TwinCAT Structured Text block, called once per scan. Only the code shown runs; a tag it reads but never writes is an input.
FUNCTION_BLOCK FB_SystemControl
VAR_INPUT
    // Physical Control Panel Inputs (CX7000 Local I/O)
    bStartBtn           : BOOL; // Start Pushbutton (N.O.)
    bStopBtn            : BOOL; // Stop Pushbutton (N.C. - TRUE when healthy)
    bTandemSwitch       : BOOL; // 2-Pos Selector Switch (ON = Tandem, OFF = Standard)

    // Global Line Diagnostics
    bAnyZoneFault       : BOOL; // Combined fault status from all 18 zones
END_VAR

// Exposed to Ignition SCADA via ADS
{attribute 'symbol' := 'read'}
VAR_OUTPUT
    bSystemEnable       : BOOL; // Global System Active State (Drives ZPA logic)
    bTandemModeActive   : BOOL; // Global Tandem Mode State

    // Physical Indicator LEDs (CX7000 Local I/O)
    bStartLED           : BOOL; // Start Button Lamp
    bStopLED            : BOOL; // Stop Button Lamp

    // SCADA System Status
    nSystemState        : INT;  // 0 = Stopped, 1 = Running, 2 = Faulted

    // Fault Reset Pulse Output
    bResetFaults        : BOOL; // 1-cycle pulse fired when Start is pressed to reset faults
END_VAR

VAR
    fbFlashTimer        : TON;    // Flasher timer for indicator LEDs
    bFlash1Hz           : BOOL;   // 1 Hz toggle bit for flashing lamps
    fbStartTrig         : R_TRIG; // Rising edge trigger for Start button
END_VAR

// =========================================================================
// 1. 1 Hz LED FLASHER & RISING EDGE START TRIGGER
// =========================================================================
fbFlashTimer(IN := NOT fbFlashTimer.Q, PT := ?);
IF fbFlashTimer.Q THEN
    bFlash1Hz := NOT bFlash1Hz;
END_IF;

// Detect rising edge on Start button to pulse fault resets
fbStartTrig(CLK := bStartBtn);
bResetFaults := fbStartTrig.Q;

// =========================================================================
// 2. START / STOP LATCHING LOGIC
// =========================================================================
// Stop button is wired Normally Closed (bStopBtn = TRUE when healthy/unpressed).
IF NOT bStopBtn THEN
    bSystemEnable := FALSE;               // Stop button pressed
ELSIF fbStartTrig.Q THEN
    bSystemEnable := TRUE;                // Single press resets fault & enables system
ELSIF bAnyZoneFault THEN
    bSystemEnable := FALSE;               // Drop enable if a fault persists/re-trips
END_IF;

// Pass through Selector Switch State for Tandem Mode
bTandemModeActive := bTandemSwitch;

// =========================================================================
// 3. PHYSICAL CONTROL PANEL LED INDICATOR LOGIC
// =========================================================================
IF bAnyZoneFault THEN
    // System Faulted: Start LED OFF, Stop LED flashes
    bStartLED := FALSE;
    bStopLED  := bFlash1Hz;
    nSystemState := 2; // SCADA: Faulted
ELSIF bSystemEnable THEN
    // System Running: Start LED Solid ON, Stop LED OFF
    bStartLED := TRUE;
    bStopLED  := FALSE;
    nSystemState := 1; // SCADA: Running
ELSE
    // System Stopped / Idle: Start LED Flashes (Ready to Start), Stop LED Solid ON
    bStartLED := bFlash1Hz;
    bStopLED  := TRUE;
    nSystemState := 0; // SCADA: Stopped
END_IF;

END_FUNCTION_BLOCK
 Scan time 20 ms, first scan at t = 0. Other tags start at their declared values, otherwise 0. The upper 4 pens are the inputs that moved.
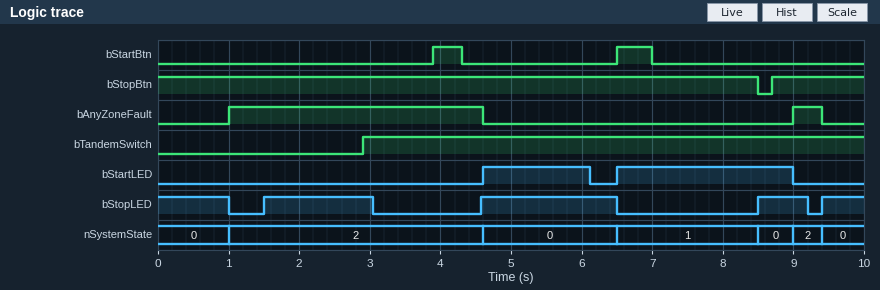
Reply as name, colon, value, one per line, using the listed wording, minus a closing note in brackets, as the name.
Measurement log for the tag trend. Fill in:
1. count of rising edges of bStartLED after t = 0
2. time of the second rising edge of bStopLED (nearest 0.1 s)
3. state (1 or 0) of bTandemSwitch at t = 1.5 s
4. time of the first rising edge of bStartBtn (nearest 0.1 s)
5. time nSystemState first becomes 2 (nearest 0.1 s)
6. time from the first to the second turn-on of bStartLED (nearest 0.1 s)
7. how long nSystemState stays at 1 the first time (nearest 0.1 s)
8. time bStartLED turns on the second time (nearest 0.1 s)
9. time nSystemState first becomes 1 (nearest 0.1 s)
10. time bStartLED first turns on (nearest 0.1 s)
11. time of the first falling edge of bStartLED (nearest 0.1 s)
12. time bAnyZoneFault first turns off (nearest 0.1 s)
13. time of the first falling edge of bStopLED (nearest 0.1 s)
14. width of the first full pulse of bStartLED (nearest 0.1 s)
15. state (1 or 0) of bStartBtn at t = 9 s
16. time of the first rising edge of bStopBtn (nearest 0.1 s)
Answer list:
count of rising edges of bStartLED after t = 0: 2
time of the second rising edge of bStopLED: 4.6 s
state (1 or 0) of bTandemSwitch at t = 1.5 s: 0
time of the first rising edge of bStartBtn: 3.9 s
time nSystemState first becomes 2: 1.0 s
time from the first to the second turn-on of bStartLED: 1.9 s
how long nSystemState stays at 1 the first time: 2.0 s
time bStartLED turns on the second time: 6.5 s
time nSystemState first becomes 1: 6.5 s
time bStartLED first turns on: 4.6 s
time of the first falling edge of bStartLED: 6.1 s
time bAnyZoneFault first turns off: 4.6 s
time of the first falling edge of bStopLED: 1.0 s
width of the first full pulse of bStartLED: 1.5 s
state (1 or 0) of bStartBtn at t = 9 s: 0
time of the first rising edge of bStopBtn: 8.7 s
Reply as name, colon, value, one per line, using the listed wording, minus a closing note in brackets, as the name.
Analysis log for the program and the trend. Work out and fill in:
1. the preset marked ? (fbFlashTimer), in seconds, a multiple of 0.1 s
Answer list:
the preset marked ? (fbFlashTimer), in seconds, a multiple of 0.1 s: 1.5 s
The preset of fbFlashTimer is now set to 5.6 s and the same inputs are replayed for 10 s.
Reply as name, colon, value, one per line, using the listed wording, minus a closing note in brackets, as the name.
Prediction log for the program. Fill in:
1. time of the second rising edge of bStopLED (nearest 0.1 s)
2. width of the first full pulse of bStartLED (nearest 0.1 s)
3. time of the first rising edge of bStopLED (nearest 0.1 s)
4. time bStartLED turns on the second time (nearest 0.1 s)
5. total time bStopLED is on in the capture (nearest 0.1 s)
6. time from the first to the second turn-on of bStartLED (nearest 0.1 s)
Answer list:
time of the second rising edge of bStopLED: 8.5 s
width of the first full pulse of bStartLED: 3.4 s
time of the first rising edge of bStopLED: 4.6 s
time bStartLED turns on the second time: 9.4 s
total time bStopLED is on in the capture: 4.4 s
time from the first to the second turn-on of bStartLED: 3.8 s
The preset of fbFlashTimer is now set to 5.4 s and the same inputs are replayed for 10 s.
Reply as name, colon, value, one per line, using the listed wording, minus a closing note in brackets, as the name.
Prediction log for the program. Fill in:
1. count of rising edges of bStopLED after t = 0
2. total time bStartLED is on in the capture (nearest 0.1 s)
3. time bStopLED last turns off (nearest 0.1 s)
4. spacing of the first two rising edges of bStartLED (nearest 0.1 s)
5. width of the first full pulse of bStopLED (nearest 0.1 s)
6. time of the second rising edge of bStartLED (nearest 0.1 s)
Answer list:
count of rising edges of bStopLED after t = 0: 2
total time bStartLED is on in the capture: 4.2 s
time bStopLED last turns off: 6.5 s
spacing of the first two rising edges of bStartLED: 4.0 s
width of the first full pulse of bStopLED: 1.9 s
time of the second rising edge of bStartLED: 9.4 s
